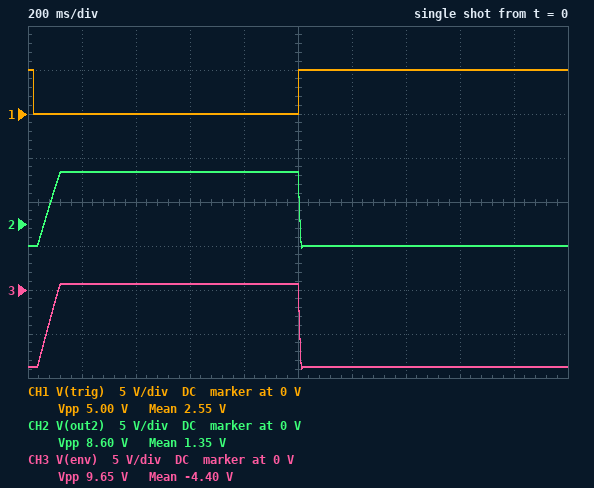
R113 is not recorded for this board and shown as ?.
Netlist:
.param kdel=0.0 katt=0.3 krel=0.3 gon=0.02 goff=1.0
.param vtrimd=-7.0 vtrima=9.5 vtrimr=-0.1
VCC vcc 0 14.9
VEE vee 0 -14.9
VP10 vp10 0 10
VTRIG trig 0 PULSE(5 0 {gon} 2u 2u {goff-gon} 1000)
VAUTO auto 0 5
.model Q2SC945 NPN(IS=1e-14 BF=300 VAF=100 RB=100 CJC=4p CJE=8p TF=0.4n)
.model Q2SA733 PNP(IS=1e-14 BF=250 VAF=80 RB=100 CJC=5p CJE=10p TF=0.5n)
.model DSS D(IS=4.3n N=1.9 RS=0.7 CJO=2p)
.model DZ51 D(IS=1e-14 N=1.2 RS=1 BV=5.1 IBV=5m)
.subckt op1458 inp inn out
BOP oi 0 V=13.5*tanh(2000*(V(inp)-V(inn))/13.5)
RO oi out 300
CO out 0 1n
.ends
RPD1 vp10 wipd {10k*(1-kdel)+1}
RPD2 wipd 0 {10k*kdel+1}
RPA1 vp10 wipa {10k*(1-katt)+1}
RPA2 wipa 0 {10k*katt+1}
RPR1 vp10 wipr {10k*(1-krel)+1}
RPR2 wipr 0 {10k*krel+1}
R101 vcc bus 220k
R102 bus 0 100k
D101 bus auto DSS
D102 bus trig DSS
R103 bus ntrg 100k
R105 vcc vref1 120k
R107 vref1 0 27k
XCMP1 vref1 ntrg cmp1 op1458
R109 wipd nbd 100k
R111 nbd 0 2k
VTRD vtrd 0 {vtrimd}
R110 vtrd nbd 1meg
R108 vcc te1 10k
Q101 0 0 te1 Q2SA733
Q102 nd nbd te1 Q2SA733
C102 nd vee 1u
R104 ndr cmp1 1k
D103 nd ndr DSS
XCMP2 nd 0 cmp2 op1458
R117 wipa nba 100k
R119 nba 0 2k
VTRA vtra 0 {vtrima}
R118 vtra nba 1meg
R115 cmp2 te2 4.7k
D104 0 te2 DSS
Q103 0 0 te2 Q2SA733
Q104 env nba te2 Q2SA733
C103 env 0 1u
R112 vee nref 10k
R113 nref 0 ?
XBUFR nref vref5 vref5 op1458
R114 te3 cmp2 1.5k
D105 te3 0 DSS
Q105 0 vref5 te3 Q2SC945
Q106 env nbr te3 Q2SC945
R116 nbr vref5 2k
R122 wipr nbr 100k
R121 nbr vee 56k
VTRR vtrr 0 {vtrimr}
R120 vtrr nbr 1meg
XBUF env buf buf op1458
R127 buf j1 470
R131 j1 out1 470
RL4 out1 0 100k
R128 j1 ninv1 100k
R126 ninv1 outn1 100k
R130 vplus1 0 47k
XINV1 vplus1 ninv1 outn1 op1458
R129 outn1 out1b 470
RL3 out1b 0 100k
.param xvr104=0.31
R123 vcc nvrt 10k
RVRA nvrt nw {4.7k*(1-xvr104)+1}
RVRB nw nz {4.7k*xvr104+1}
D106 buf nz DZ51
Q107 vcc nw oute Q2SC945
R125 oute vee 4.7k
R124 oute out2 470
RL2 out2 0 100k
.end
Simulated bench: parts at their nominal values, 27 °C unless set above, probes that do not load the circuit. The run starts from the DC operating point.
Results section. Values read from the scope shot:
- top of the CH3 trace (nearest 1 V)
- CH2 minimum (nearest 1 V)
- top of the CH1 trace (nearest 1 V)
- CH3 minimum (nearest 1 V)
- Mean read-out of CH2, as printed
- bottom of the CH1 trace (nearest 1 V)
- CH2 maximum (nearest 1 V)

1 V
-3 V
5 V
-9 V
1.35 V
0 V
6 V
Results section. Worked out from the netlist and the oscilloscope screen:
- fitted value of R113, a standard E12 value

12 kΩ
